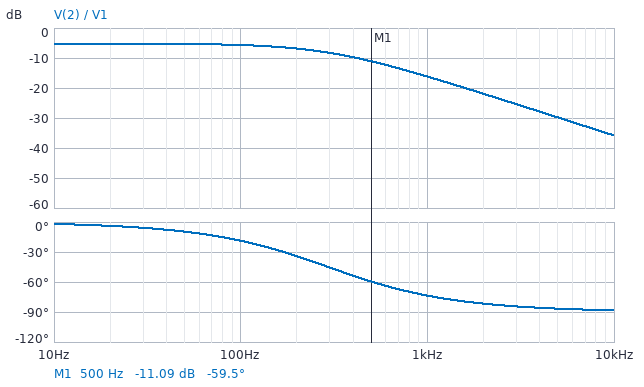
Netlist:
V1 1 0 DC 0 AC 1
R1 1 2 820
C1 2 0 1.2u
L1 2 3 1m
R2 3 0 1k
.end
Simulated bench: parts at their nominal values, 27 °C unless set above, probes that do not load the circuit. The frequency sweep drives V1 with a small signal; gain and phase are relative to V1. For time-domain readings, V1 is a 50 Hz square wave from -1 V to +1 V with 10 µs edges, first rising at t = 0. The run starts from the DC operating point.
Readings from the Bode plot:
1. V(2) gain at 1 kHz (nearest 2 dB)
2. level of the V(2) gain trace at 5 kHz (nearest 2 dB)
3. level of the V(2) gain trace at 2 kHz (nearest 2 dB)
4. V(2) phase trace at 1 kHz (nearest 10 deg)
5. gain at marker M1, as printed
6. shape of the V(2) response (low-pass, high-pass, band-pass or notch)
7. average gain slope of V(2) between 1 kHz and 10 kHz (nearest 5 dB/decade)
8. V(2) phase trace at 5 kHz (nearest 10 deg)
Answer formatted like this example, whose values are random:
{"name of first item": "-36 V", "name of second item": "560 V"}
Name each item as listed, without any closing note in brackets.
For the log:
{"V(2) gain at 1 kHz": "-16 dB", "level of the V(2) gain trace at 5 kHz": "-30 dB", "level of the V(2) gain trace at 2 kHz": "-22 dB", "V(2) phase trace at 1 kHz": "-70 deg", "gain at marker M1, as printed": "-11.09 dB", "shape of the V(2) response": "low-pass", "average gain slope of V(2) between 1 kHz and 10 kHz": "-20 dB/decade", "V(2) phase trace at 5 kHz": "-90 deg"}
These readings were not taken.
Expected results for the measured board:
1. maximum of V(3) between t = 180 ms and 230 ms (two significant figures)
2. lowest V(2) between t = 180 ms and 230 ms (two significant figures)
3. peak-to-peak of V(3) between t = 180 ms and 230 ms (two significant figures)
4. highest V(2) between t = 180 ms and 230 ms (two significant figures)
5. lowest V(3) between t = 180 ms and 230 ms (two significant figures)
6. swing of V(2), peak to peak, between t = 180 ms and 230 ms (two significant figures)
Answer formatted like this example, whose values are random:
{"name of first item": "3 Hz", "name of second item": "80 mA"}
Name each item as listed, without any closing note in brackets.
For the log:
{"maximum of V(3) between t = 180 ms and 230 ms": "550 mV", "lowest V(2) between t = 180 ms and 230 ms": "-550 mV", "peak-to-peak of V(3) between t = 180 ms and 230 ms": "1.1 V", "highest V(2) between t = 180 ms and 230 ms": "550 mV", "lowest V(3) between t = 180 ms and 230 ms": "-550 mV", "swing of V(2), peak to peak, between t = 180 ms and 230 ms": "1.1 V"}
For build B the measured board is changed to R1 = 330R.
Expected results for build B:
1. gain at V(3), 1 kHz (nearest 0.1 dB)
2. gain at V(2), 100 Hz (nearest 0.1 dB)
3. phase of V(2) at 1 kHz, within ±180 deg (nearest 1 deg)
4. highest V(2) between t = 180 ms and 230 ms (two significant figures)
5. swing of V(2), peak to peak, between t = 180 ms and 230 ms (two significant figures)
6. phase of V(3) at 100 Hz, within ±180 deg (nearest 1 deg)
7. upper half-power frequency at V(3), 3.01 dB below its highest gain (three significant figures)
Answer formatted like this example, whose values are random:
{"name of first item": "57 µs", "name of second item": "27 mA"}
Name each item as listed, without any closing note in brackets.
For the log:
{"gain at V(3), 1 kHz": "-9.0 dB", "gain at V(2), 100 Hz": "-2.6 dB", "phase of V(2) at 1 kHz, within ±180 deg": "-62 deg", "highest V(2) between t = 180 ms and 230 ms": "750 mV", "swing of V(2), peak to peak, between t = 180 ms and 230 ms": "1.5 V", "phase of V(3) at 100 Hz, within ±180 deg": "-11 deg", "upper half-power frequency at V(3), 3.01 dB below its highest gain": "535 Hz"}
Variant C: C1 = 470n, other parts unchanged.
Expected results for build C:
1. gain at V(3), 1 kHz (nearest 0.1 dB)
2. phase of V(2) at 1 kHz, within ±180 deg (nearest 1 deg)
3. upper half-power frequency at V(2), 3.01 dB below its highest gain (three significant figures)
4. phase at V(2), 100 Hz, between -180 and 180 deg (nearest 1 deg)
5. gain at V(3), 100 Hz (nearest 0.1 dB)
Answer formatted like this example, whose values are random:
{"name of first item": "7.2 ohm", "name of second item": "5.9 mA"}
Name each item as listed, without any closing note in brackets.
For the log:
{"gain at V(3), 1 kHz": "-9.6 dB", "phase of V(2) at 1 kHz, within ±180 deg": "-53 deg", "upper half-power frequency at V(2), 3.01 dB below its highest gain": "753 Hz", "phase at V(2), 100 Hz, between -180 and 180 deg": "-8 deg", "gain at V(3), 100 Hz": "-5.3 dB"}
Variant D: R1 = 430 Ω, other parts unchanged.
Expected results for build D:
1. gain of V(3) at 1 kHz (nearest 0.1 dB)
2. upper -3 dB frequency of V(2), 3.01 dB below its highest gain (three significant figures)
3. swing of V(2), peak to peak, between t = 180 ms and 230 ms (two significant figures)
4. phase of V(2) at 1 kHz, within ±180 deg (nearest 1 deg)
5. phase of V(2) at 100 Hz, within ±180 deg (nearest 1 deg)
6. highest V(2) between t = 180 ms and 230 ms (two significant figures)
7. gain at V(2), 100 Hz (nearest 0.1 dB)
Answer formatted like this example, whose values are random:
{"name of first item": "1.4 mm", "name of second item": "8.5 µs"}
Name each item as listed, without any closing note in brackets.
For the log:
{"gain of V(3) at 1 kHz": "-11.0 dB", "upper -3 dB frequency of V(2), 3.01 dB below its highest gain": "441 Hz", "swing of V(2), peak to peak, between t = 180 ms and 230 ms": "1.4 V", "phase of V(2) at 1 kHz, within ±180 deg": "-66 deg", "phase of V(2) at 100 Hz, within ±180 deg": "-13 deg", "highest V(2) between t = 180 ms and 230 ms": "700 mV", "gain at V(2), 100 Hz": "-3.3 dB"}
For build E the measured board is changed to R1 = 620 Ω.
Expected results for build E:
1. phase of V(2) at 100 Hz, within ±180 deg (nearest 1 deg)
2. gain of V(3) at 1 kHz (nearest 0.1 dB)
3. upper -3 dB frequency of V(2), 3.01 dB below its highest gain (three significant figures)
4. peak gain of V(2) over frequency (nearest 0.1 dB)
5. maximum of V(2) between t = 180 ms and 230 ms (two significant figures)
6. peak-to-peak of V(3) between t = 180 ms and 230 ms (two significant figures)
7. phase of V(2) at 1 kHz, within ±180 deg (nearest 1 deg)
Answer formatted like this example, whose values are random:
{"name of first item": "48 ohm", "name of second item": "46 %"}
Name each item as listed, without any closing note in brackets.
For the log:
{"phase of V(2) at 100 Hz, within ±180 deg": "-16 deg", "gain of V(3) at 1 kHz": "-13.9 dB", "upper -3 dB frequency of V(2), 3.01 dB below its highest gain": "347 Hz", "peak gain of V(2) over frequency": "-4.2 dB", "maximum of V(2) between t = 180 ms and 230 ms": "620 mV", "peak-to-peak of V(3) between t = 180 ms and 230 ms": "1.2 V", "phase of V(2) at 1 kHz, within ±180 deg": "-71 deg"}
